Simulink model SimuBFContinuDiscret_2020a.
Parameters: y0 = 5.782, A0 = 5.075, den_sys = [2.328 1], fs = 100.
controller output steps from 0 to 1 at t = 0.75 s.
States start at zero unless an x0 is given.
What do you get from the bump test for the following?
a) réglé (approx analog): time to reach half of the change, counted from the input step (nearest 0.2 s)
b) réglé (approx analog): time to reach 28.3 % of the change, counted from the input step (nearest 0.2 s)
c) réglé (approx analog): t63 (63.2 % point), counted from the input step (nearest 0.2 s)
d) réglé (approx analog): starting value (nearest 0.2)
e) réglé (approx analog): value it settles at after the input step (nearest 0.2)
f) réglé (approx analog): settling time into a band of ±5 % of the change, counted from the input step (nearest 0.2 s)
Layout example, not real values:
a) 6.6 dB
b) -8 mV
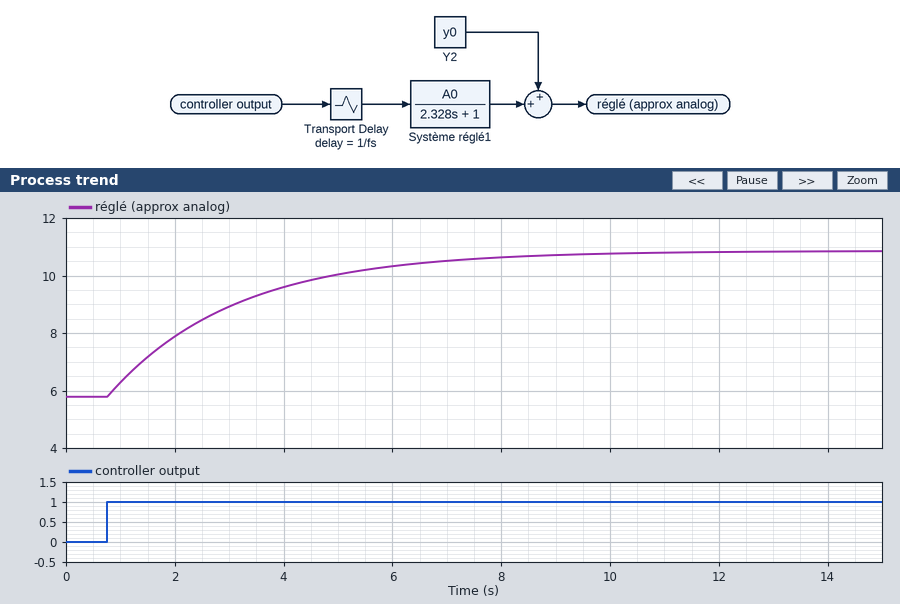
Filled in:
a) 1.6 s
b) 0.8 s
c) 2.4 s
d) 5.8
e) 10.8
f) 7.0 s
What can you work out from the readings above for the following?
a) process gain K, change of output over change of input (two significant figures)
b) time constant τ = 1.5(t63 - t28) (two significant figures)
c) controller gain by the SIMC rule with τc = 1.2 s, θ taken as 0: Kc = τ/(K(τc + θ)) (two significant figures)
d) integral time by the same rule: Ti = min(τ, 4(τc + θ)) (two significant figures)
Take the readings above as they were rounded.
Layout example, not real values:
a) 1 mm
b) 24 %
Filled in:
a) 5.0
b) 2.4 s
c) 0.40
d) 2.4 s
